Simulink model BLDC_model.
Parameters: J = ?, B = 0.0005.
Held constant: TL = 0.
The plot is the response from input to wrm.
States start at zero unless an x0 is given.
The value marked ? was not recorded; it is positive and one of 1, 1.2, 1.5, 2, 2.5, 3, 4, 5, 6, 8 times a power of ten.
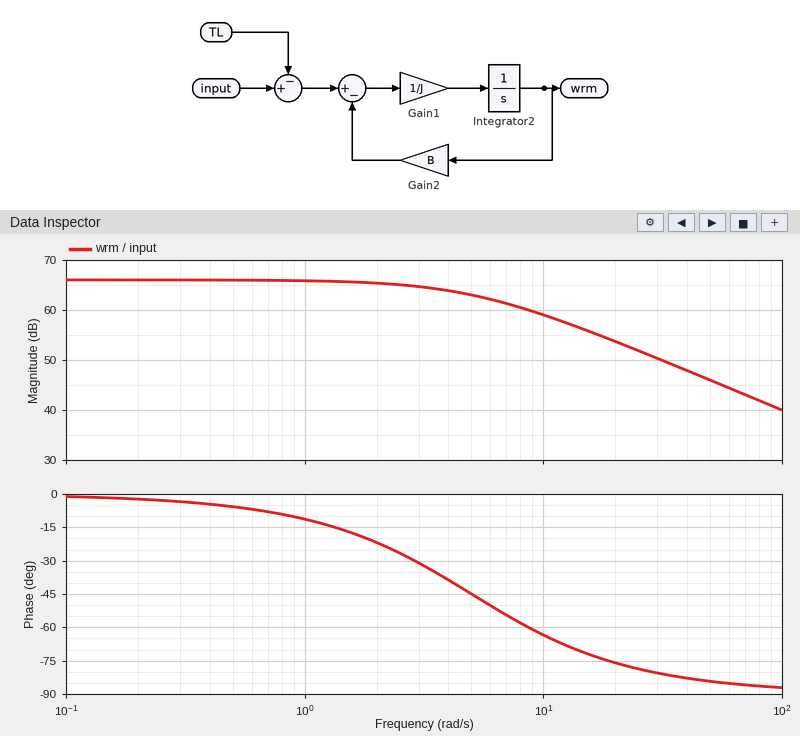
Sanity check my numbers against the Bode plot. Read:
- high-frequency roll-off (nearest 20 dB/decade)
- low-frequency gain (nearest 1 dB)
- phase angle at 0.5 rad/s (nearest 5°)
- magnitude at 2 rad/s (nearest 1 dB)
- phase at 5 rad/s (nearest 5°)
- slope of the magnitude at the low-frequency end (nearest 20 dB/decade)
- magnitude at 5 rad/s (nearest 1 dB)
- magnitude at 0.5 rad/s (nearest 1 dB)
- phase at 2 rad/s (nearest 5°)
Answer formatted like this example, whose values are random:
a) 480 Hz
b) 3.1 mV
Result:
a) -20 dB/decade
b) 66 dB
c) -5°
d) 65 dB
e) -45°
f) 0 dB/decade
g) 63 dB
h) 66 dB
i) -20°
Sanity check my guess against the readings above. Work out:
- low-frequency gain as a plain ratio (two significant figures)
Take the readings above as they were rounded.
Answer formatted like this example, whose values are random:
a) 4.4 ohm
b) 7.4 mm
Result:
a) 2000
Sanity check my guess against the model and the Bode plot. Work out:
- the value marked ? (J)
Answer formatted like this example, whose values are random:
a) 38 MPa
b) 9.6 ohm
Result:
a) 0.0001
